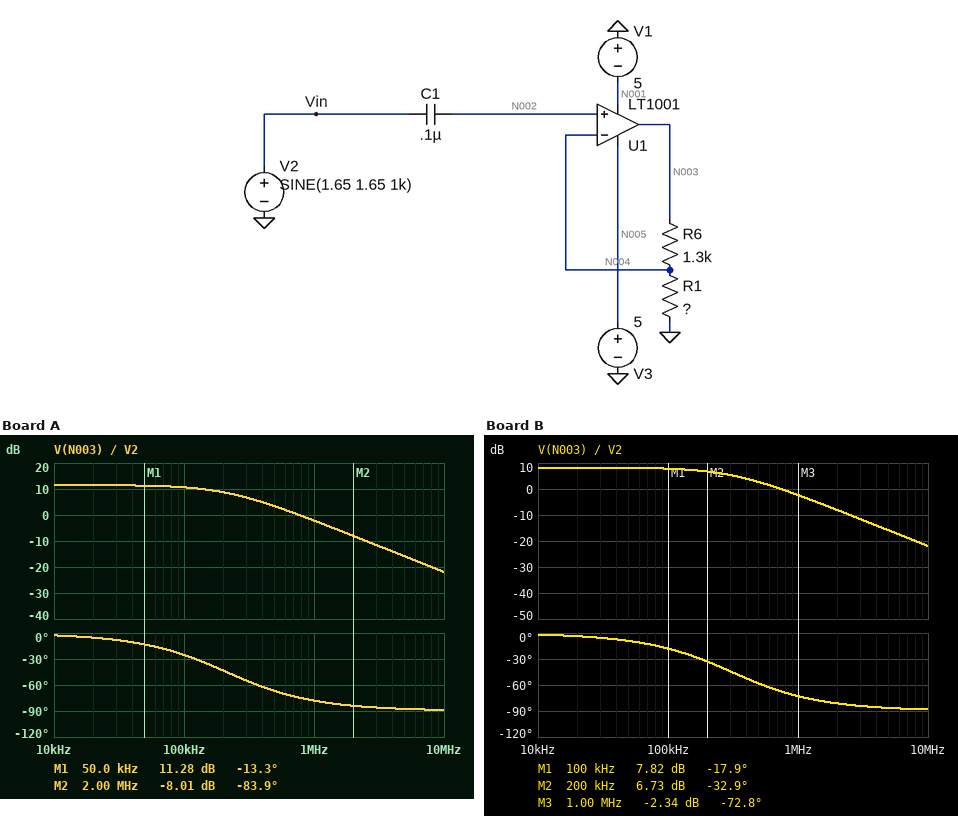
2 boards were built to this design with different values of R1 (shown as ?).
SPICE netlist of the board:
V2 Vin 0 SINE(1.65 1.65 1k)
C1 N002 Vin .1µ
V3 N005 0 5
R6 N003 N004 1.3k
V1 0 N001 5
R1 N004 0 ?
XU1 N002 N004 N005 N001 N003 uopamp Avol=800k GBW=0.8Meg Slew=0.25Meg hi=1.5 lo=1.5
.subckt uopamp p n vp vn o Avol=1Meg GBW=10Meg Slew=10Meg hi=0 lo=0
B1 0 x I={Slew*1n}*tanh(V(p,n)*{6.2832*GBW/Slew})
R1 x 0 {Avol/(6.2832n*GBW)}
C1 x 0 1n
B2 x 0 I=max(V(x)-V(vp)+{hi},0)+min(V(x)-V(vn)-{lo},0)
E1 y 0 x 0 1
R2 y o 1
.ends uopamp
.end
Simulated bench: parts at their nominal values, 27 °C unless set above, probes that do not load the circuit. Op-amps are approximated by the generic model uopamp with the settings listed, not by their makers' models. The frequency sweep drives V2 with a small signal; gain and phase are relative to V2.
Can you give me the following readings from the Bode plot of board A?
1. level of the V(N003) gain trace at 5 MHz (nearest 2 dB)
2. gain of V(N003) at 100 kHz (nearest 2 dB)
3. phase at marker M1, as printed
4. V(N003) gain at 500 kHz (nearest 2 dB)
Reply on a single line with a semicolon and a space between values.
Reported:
-16 dB; 10 dB; -13.3 deg; 4 dB
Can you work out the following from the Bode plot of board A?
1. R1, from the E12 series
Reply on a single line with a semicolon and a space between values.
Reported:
470 Ω
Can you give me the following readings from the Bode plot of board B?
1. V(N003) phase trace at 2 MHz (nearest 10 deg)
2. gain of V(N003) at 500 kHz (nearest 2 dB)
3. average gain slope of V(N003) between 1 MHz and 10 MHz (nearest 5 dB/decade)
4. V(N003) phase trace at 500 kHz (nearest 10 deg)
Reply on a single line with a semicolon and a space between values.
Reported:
-80 deg; 2 dB; -20 dB/decade; -60 deg
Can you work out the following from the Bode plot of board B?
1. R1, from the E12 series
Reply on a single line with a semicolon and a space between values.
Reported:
820 Ω
